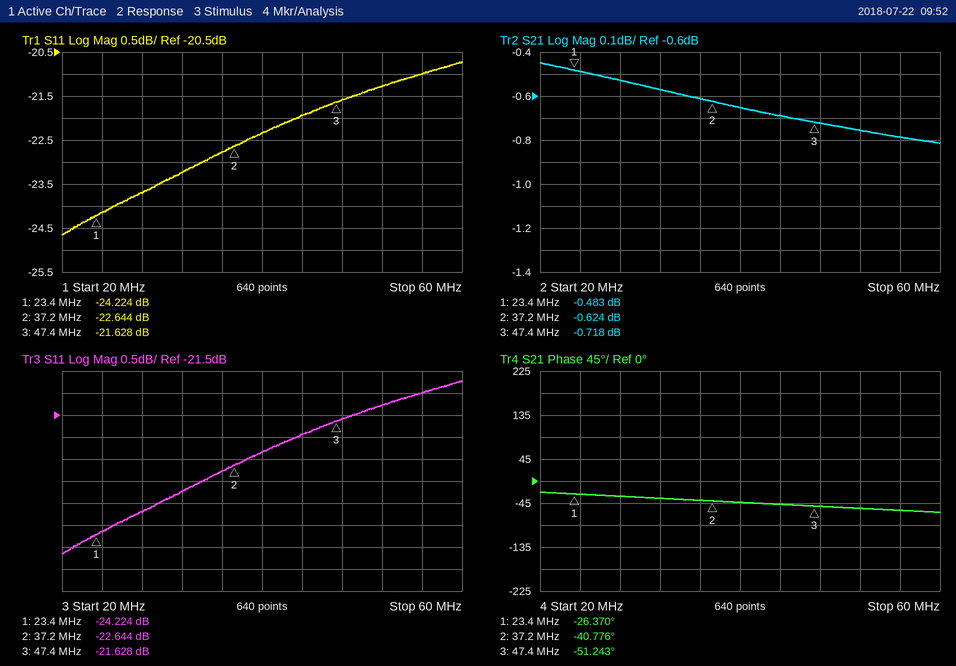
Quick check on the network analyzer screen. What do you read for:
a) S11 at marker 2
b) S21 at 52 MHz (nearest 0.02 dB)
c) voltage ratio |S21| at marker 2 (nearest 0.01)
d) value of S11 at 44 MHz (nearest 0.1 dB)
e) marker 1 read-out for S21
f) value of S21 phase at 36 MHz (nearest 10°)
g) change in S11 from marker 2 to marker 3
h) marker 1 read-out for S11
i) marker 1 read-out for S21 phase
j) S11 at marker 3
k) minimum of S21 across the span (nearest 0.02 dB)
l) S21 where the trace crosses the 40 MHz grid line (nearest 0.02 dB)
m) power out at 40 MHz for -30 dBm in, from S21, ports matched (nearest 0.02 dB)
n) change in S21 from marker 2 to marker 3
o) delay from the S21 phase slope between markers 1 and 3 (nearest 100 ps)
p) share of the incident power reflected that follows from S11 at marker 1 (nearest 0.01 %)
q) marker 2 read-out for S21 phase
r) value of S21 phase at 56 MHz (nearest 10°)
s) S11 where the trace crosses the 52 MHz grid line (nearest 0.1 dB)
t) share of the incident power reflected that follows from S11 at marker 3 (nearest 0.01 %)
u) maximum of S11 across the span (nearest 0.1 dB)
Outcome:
-22.644 dB
-0.76 dB
0.93
-21.9 dB
-0.483 dB
-40°
1.016 dB
-24.224 dB
-26.370°
-21.628 dB
-0.82 dB
-0.66 dB
-30.66 dBm
-0.094 dB
2.9 ns
0.38 %
-40.776°
-60°
-21.3 dB
0.69 %
-20.7 dB
